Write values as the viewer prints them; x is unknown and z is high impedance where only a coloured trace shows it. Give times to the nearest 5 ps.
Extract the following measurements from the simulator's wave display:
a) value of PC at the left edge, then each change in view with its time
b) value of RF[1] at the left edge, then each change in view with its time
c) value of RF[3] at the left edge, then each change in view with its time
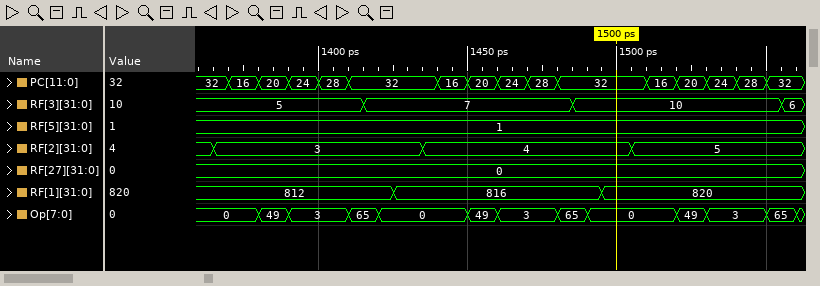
32, 16 at 1370 ps, 20 at 1380 ps, 24 at 1390 ps, 28 at 1400 ps, 32 at 1410 ps, 16 at 1440 ps, 20 at 1450 ps, 24 at 1460 ps, 28 at 1470 ps, 32 at 1480 ps, 16 at 1510 ps, 20 at 1520 ps, 24 at 1530 ps, 28 at 1540 ps, 32 at 1550 ps
812, 816 at 1425 ps, 820 at 1495 ps
5, 7 at 1415 ps, 10 at 1485 ps, 6 at 1555 ps
